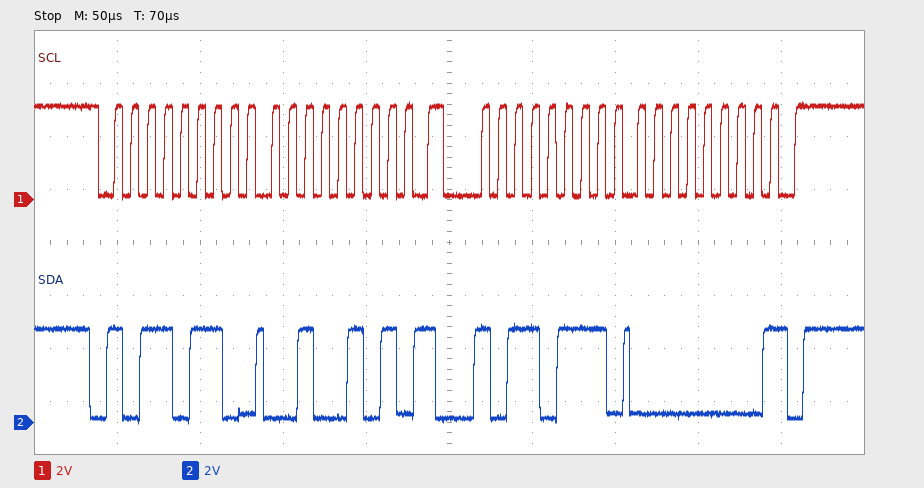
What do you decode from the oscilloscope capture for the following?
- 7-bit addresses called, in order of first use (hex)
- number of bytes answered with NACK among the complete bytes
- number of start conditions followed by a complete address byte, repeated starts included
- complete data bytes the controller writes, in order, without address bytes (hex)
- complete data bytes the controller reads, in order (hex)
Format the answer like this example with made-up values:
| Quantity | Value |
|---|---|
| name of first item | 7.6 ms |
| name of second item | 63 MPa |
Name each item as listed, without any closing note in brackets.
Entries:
| Quantity | Value |
|---|---|
| 7-bit addresses called, in order of first use | 0x5B |
| number of bytes answered with NACK among the complete bytes | 1 |
| number of start conditions followed by a complete address byte, repeated starts included | 2 |
| complete data bytes the controller writes, in order, without address bytes | 25 |
| complete data bytes the controller reads, in order | 00 |
